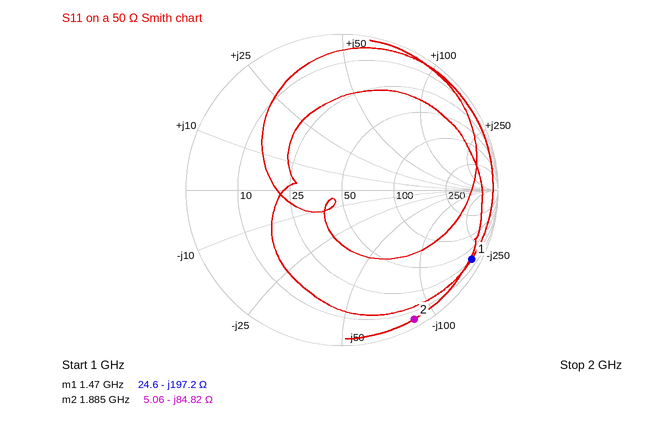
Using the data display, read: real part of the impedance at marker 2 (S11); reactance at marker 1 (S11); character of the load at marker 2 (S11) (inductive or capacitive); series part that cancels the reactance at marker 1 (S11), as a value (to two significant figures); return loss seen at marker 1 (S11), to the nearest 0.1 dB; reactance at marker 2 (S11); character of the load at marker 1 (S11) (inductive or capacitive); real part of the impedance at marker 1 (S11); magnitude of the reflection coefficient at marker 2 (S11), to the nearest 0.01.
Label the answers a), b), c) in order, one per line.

a) 5.06 Ω
b) -197.2 Ω
c) capacitive
d) 21 nH
e) 0.5 dB
f) -84.82 Ω
g) capacitive
h) 24.6 Ω
i) 0.95
